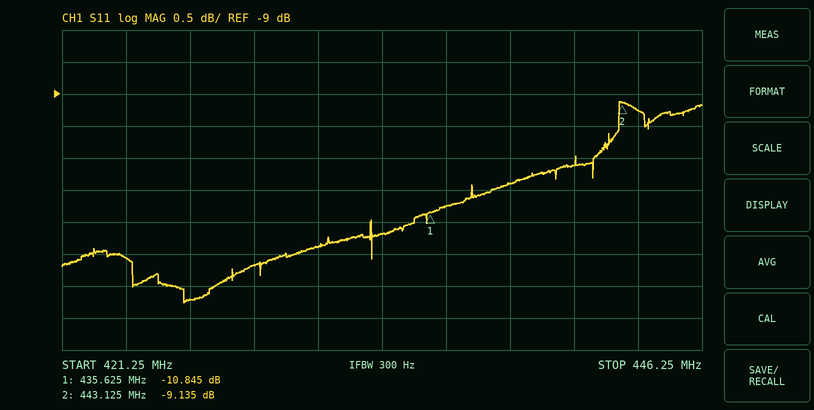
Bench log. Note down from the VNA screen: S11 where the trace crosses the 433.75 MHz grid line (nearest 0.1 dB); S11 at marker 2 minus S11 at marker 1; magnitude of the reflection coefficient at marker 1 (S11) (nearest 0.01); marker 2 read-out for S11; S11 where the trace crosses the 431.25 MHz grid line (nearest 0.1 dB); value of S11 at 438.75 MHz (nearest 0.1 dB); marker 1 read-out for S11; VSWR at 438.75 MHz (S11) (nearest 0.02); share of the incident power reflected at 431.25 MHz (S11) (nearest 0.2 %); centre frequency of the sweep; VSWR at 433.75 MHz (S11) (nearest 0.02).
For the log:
-11.2 dB
1.710 dB
0.29
-9.135 dB
-11.4 dB
-10.4 dB
-10.845 dB
1.86
7.2 %
433.75 MHz
1.76
